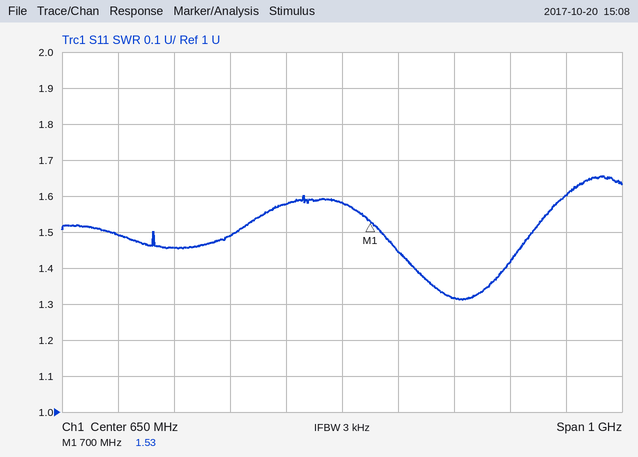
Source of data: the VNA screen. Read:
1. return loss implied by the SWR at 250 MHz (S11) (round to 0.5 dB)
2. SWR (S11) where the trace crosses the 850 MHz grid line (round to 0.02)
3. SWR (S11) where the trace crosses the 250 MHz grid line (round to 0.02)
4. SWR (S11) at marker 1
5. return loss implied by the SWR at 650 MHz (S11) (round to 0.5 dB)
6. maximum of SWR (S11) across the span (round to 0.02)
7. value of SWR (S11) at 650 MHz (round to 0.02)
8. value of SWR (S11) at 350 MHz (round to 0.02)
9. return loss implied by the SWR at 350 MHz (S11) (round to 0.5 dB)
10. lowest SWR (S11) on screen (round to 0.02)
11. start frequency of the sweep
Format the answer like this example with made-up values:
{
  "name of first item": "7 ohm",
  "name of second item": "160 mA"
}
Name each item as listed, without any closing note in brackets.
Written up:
{
  "return loss implied by the SWR at 250 MHz (S11)": "14.0 dB",
  "SWR (S11) where the trace crosses the 850 MHz grid line": "1.32",
  "SWR (S11) where the trace crosses the 250 MHz grid line": "1.50",
  "SWR (S11) at marker 1": "1.53",
  "return loss implied by the SWR at 650 MHz (S11)": "13.0 dB",
  "maximum of SWR (S11) across the span": "1.66",
  "value of SWR (S11) at 650 MHz": "1.58",
  "value of SWR (S11) at 350 MHz": "1.46",
  "return loss implied by the SWR at 350 MHz (S11)": "14.5 dB",
  "lowest SWR (S11) on screen": "1.32",
  "start frequency of the sweep": "150 MHz"
}
